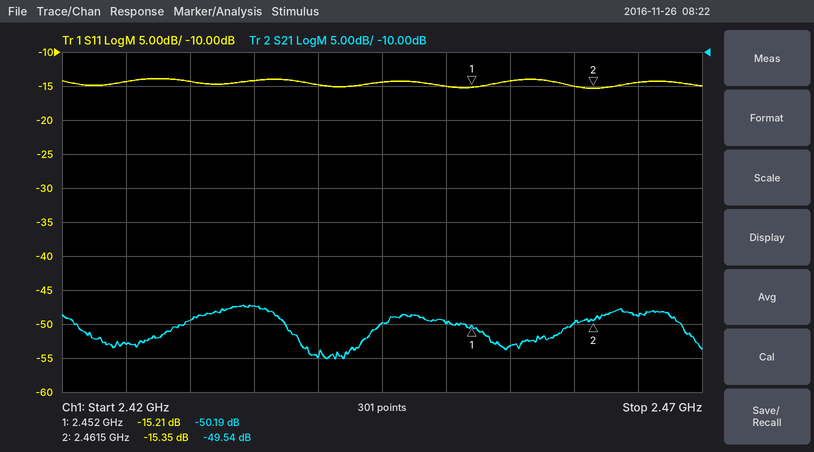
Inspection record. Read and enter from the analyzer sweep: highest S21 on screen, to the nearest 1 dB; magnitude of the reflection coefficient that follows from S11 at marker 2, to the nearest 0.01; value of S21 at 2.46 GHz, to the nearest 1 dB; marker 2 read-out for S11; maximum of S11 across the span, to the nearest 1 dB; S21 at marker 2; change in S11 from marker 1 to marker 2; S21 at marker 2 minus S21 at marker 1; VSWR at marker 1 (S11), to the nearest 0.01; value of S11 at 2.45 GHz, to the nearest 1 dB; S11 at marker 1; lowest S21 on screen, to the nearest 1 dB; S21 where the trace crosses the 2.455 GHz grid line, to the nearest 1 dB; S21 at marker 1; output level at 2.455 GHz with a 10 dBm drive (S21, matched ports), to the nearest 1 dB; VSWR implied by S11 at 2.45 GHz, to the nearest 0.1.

-47 dB
0.17
-50 dB
-15.35 dB
-14 dB
-49.54 dB
-0.14 dB
0.65 dB
1.42
-15 dB
-15.21 dB
-55 dB
-53 dB
-50.19 dB
-43 dBm
1.4
